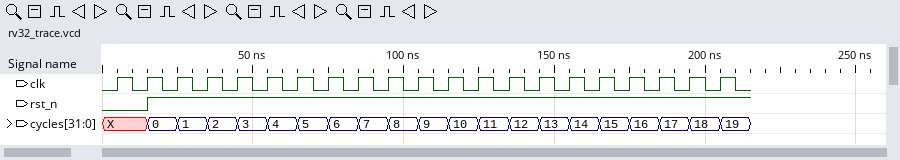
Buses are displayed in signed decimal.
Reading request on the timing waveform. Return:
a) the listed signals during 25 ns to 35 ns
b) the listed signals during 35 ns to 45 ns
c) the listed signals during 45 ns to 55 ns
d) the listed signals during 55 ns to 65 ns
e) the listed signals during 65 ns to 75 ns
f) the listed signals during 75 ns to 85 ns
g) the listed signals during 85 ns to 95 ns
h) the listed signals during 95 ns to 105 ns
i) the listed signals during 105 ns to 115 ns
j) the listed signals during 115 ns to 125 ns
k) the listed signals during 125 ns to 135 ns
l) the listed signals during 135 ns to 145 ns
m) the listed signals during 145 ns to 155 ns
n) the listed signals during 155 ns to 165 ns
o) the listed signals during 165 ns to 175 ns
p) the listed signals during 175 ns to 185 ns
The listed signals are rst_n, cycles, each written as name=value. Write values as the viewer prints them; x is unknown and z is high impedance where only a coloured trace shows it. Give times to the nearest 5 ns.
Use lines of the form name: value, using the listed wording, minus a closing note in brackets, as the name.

the listed signals during 25 ns to 35 ns: rst_n=1, cycles=1
the listed signals during 35 ns to 45 ns: rst_n=1, cycles=2
the listed signals during 45 ns to 55 ns: rst_n=1, cycles=3
the listed signals during 55 ns to 65 ns: rst_n=1, cycles=4
the listed signals during 65 ns to 75 ns: rst_n=1, cycles=5
the listed signals during 75 ns to 85 ns: rst_n=1, cycles=6
the listed signals during 85 ns to 95 ns: rst_n=1, cycles=7
the listed signals during 95 ns to 105 ns: rst_n=1, cycles=8
the listed signals during 105 ns to 115 ns: rst_n=1, cycles=9
the listed signals during 115 ns to 125 ns: rst_n=1, cycles=10
the listed signals during 125 ns to 135 ns: rst_n=1, cycles=11
the listed signals during 135 ns to 145 ns: rst_n=1, cycles=12
the listed signals during 145 ns to 155 ns: rst_n=1, cycles=13
the listed signals during 155 ns to 165 ns: rst_n=1, cycles=14
the listed signals during 165 ns to 175 ns: rst_n=1, cycles=15
the listed signals during 175 ns to 185 ns: rst_n=1, cycles=16
